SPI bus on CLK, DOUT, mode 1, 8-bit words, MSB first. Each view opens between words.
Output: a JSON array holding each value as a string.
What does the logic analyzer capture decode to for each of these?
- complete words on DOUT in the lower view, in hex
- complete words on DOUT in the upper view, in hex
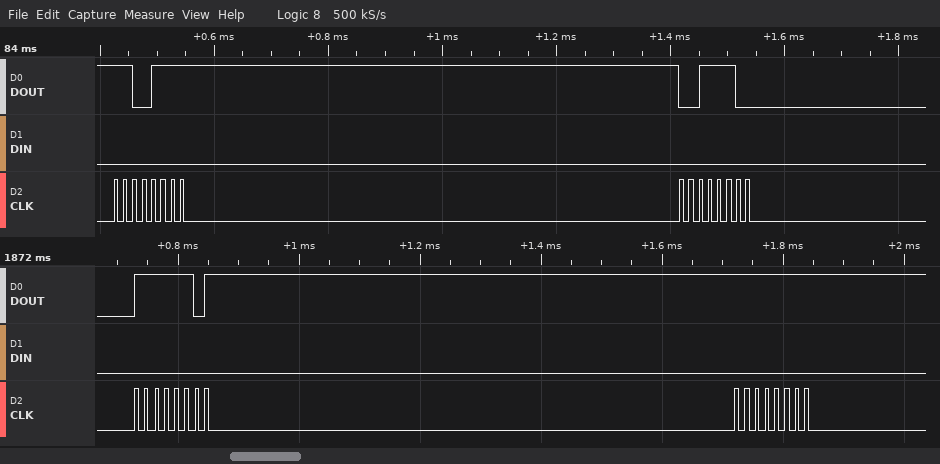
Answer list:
["FD, FF", "CF, 3C"]
